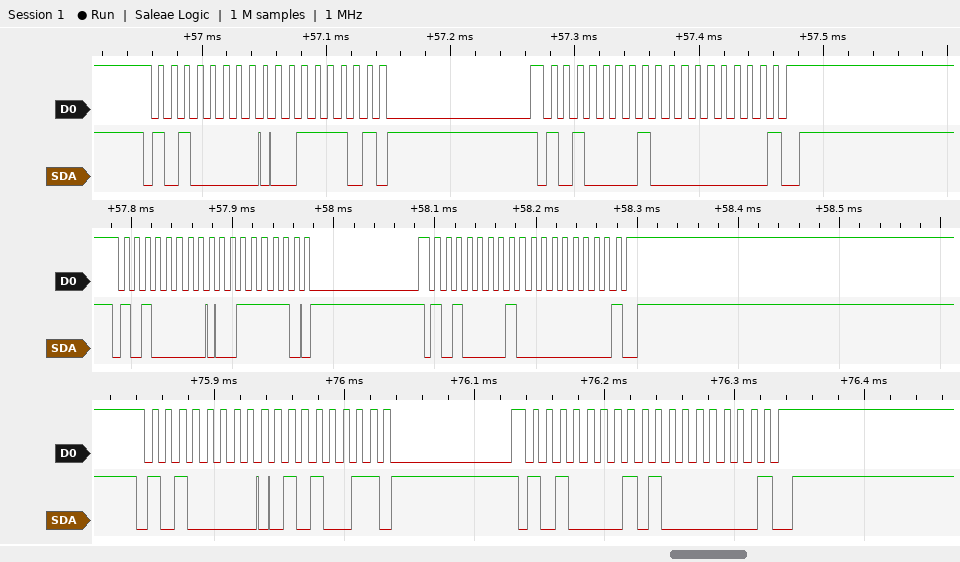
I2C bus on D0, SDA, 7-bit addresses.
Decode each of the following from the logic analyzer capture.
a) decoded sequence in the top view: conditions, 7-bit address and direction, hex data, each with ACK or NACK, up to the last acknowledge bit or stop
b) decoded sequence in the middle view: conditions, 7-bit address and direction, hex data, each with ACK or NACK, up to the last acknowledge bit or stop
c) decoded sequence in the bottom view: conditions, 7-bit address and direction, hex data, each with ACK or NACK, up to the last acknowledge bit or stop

start, address 50 write ACK, 3D ACK, repeated start, address 50 read ACK, 00 NACK, stop
start, address 50 write ACK, 3E ACK, repeated start, address 50 read ACK, 00 NACK, stop
start, address 50 write ACK, 53 ACK, repeated start, address 50 read ACK, 80 NACK, stop
